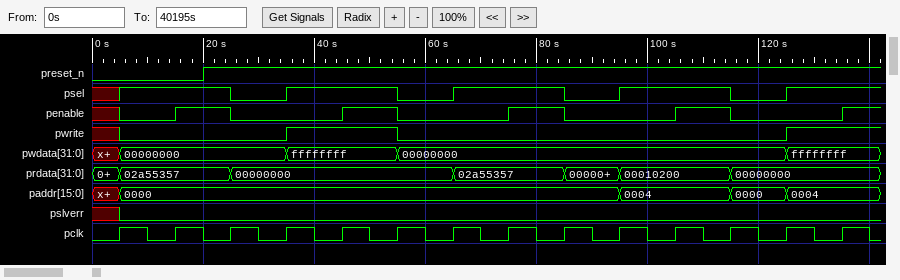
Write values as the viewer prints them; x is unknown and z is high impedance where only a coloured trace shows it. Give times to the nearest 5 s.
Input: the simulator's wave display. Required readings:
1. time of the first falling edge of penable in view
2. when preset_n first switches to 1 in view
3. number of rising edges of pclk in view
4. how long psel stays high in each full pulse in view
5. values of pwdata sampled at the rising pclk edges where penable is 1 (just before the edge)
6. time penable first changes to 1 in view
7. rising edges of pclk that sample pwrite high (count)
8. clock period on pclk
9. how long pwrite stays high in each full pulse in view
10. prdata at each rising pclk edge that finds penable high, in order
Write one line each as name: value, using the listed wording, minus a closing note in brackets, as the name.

time of the first falling edge of penable in view: 25 s
when preset_n first switches to 1 in view: 20 s
number of rising edges of pclk in view: 14
how long psel stays high in each full pulse in view: 20 s, 20 s, 20 s
values of pwdata sampled at the rising pclk edges where penable is 1: 00000000, ffffffff, 00000000, 00000000
time penable first changes to 1 in view: 15 s
rising edges of pclk that sample pwrite high: 3
clock period on pclk: 10 s
how long pwrite stays high in each full pulse in view: 20 s
prdata at each rising pclk edge that finds penable high, in order: 02a55357, 00000000, 02a55357, 00010200
